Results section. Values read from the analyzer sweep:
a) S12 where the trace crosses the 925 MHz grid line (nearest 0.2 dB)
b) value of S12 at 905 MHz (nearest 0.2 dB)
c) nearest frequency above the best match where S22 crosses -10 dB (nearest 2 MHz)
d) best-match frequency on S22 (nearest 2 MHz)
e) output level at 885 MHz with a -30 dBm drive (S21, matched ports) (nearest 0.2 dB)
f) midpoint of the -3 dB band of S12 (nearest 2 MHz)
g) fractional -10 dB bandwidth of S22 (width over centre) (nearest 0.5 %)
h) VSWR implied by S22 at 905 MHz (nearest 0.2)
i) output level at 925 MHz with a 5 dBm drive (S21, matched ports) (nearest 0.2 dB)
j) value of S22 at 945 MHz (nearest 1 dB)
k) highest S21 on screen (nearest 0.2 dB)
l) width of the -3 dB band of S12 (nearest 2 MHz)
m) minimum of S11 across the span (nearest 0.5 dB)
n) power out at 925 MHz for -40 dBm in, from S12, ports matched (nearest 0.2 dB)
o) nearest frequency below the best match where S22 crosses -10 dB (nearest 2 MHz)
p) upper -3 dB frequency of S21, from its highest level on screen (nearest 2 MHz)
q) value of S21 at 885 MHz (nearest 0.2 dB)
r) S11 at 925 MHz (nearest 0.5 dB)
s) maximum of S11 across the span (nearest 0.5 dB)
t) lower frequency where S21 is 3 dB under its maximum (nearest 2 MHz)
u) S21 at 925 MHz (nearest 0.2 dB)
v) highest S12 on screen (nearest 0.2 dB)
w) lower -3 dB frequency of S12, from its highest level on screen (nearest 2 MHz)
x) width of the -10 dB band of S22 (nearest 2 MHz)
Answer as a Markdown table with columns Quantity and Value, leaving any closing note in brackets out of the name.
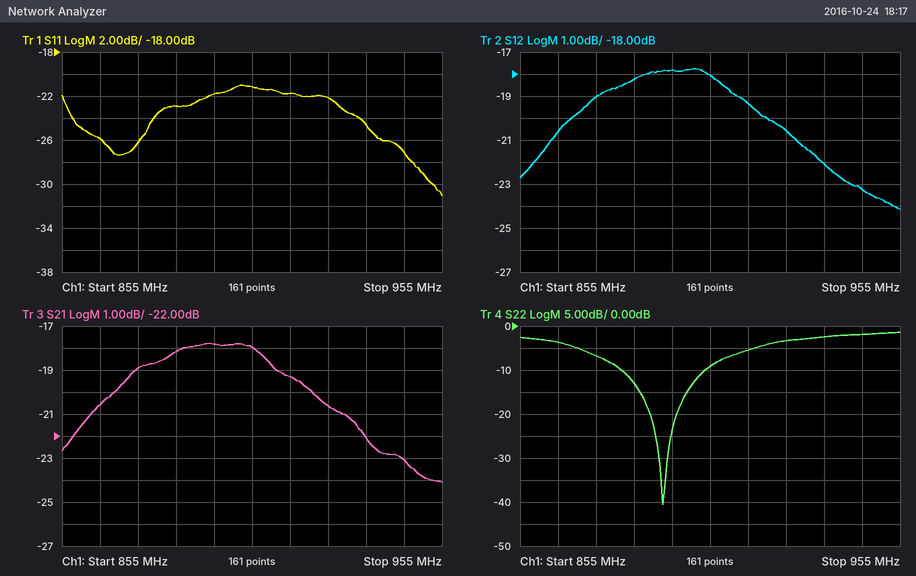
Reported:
| Quantity | Value |
|---|---|
| S12 where the trace crosses the 925 MHz grid line | -20.6 dB |
| value of S12 at 905 MHz | -18.0 dB |
| nearest frequency above the best match where S22 crosses -10 dB | 904 MHz |
| best-match frequency on S22 | 892 MHz |
| output level at 885 MHz with a -30 dBm drive (S21, matched ports) | -48.2 dBm |
| midpoint of the -3 dB band of S12 | 896 MHz |
| fractional -10 dB bandwidth of S22 (width over centre) | 2.5 % |
| VSWR implied by S22 at 905 MHz | 2.0 |
| output level at 925 MHz with a 5 dBm drive (S21, matched ports) | -15.6 dBm |
| value of S22 at 945 MHz | -2 dB |
| highest S21 on screen | -17.8 dB |
| width of the -3 dB band of S12 | 62 MHz |
| minimum of S11 across the span | -31.0 dB |
| power out at 925 MHz for -40 dBm in, from S12, ports matched | -60.6 dBm |
| nearest frequency below the best match where S22 crosses -10 dB | 882 MHz |
| upper -3 dB frequency of S21, from its highest level on screen | 926 MHz |
| value of S21 at 885 MHz | -18.2 dB |
| S11 at 925 MHz | -22.0 dB |
| maximum of S11 across the span | -21.0 dB |
| lower frequency where S21 is 3 dB under its maximum | 864 MHz |
| S21 at 925 MHz | -20.6 dB |
| highest S12 on screen | -17.8 dB |
| lower -3 dB frequency of S12, from its highest level on screen | 864 MHz |
| width of the -10 dB band of S22 | 22 MHz |
